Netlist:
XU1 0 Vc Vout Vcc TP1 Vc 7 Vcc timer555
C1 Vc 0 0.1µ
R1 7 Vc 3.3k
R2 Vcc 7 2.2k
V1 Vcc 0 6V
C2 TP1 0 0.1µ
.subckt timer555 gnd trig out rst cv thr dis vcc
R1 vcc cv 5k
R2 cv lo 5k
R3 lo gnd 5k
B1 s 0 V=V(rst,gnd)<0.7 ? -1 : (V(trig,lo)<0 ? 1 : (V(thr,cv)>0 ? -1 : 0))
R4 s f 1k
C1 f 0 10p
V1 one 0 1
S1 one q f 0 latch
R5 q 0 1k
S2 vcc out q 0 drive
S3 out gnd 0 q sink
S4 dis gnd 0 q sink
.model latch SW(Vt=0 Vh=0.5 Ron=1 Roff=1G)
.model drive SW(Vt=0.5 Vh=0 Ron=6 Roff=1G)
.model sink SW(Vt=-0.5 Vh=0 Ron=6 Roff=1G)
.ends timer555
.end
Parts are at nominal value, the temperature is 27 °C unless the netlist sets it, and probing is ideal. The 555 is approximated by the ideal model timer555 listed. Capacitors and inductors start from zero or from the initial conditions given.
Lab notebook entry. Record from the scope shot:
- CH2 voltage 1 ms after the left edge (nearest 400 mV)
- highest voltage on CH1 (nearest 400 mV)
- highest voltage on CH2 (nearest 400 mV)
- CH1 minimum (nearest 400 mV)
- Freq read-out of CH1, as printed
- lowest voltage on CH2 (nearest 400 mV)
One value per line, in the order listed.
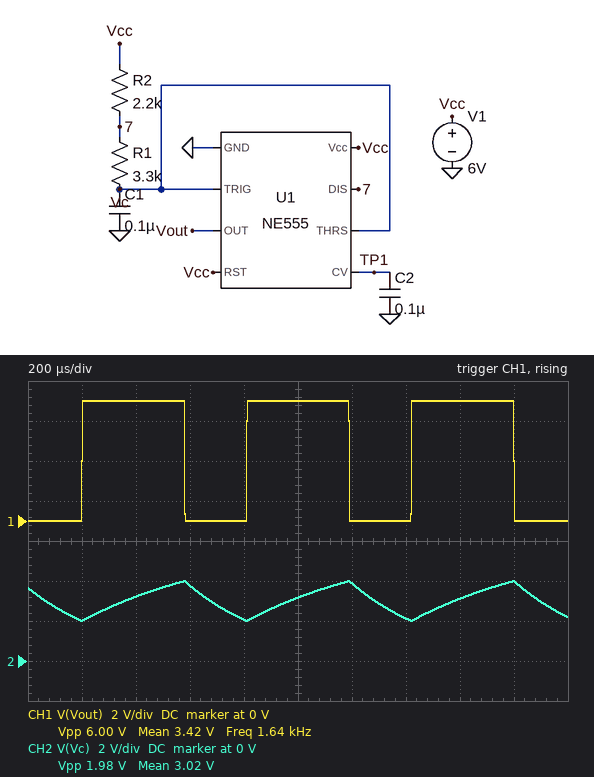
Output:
3.2 V
6.0 V
4.0 V
0 V
1.64 kHz
2.0 V
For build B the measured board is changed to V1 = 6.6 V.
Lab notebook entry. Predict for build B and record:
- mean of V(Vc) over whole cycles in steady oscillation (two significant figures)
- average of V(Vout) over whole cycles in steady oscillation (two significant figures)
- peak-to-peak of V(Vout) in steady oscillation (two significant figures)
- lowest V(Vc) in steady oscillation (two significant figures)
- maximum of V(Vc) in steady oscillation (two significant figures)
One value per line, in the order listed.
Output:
3.3 V
4.1 V
6.6 V
2.2 V
4.4 V
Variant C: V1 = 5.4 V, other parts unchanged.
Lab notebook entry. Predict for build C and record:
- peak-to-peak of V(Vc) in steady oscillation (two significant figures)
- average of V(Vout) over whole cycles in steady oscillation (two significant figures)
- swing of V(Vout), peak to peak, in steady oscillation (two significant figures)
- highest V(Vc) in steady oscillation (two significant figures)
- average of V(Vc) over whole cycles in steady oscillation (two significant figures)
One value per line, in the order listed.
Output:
1.8 V
3.4 V
5.4 V
3.6 V
2.7 V
